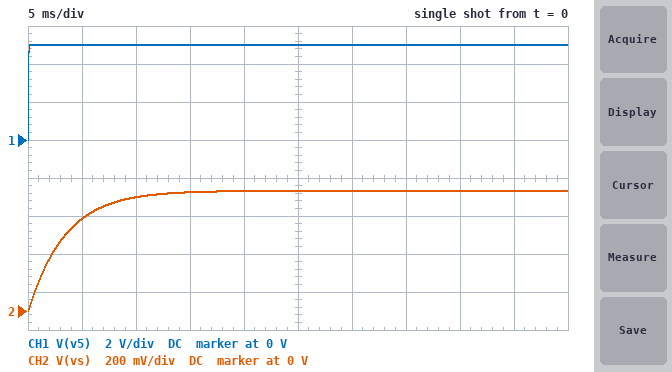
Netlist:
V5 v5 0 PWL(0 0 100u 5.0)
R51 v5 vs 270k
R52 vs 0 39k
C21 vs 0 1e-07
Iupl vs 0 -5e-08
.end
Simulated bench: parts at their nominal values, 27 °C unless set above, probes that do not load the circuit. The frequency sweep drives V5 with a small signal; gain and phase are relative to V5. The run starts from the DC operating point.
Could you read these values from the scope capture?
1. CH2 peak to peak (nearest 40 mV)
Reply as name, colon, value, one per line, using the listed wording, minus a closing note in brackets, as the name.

CH2 peak to peak: 640 mV
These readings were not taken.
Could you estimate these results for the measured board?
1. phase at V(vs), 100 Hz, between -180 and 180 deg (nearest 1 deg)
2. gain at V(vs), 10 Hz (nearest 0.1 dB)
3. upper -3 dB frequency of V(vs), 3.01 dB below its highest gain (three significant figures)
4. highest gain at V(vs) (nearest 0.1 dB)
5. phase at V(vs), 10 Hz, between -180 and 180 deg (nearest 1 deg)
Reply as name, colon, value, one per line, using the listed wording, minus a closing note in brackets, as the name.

phase at V(vs), 100 Hz, between -180 and 180 deg: -65 deg
gain at V(vs), 10 Hz: -18.2 dB
upper -3 dB frequency of V(vs), 3.01 dB below its highest gain: 46.7 Hz
highest gain at V(vs): -18.0 dB
phase at V(vs), 10 Hz, between -180 and 180 deg: -12 deg
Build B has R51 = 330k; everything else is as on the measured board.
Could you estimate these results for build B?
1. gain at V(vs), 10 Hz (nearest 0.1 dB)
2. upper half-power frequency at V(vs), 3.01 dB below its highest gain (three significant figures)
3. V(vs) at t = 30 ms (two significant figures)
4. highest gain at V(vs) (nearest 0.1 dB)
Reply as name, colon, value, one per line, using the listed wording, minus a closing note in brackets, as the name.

gain at V(vs), 10 Hz: -19.7 dB
upper half-power frequency at V(vs), 3.01 dB below its highest gain: 45.6 Hz
V(vs) at t = 30 ms: 530 mV
highest gain at V(vs): -19.5 dB
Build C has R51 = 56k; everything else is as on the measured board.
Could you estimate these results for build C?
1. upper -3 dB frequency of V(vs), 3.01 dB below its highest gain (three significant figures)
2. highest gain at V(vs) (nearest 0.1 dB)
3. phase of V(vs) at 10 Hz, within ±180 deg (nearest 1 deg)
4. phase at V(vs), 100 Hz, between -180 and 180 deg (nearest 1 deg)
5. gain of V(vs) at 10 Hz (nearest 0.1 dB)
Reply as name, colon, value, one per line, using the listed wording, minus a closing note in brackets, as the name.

upper -3 dB frequency of V(vs), 3.01 dB below its highest gain: 69.2 Hz
highest gain at V(vs): -7.7 dB
phase of V(vs) at 10 Hz, within ±180 deg: -8 deg
phase at V(vs), 100 Hz, between -180 and 180 deg: -55 deg
gain of V(vs) at 10 Hz: -7.8 dB
